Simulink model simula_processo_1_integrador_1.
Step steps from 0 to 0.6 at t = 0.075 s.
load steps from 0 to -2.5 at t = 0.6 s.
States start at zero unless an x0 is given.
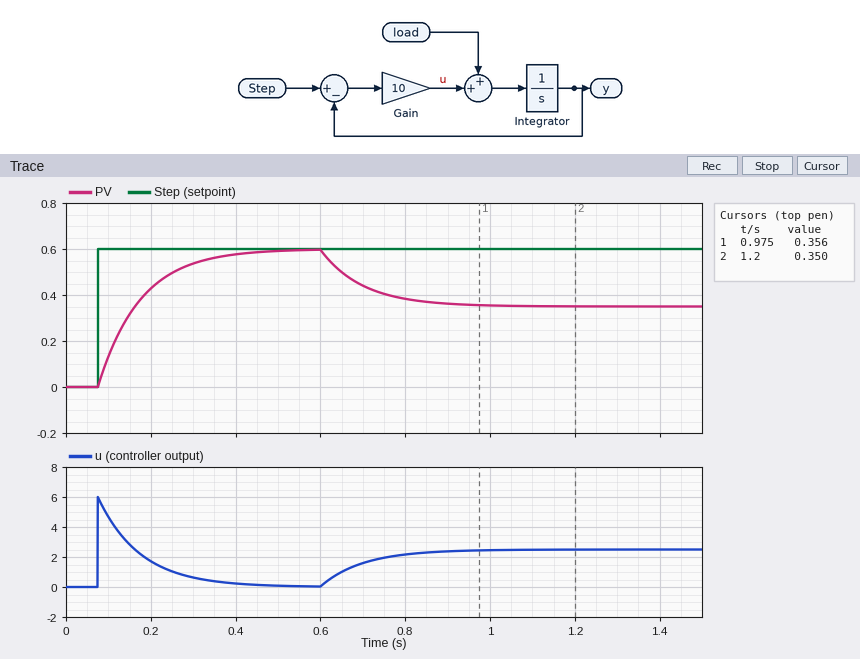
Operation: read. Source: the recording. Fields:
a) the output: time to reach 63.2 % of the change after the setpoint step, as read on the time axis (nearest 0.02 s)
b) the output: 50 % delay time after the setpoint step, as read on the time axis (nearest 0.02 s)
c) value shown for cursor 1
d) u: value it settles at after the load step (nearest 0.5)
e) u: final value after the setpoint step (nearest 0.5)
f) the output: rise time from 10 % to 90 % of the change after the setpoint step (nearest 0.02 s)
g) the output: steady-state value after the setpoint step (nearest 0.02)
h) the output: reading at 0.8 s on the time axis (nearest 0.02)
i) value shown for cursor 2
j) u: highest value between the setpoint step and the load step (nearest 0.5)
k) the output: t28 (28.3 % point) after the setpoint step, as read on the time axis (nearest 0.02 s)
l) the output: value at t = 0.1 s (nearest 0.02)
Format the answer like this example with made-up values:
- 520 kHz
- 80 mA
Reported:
- 0.18 s
- 0.14 s
- 0.356
- 2.5
- 0.0
- 0.22 s
- 0.60
- 0.38
- 0.350
- 6.0
- 0.10 s
- 0.14
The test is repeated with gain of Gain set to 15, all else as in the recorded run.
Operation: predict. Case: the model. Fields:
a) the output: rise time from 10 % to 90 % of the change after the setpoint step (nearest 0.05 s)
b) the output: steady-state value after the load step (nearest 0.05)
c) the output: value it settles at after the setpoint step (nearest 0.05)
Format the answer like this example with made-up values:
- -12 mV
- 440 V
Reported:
- 0.15 s
- 0.45
- 0.60
